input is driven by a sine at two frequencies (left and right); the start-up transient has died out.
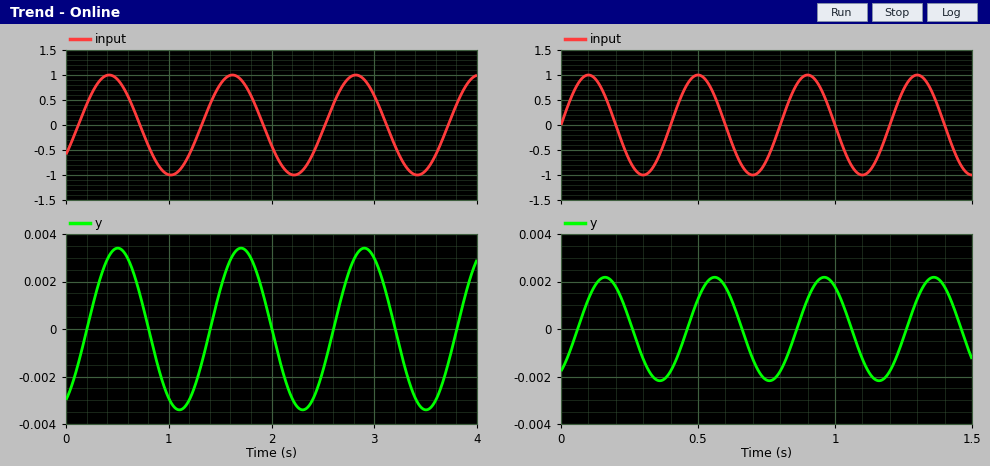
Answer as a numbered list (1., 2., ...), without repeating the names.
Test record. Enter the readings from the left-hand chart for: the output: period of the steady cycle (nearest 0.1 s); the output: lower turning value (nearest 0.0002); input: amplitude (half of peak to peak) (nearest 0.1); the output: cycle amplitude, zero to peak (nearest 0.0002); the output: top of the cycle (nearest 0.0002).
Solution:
1. 1.2 s
2. -0.0034
3. 1.0
4. 0.0034
5. 0.0034
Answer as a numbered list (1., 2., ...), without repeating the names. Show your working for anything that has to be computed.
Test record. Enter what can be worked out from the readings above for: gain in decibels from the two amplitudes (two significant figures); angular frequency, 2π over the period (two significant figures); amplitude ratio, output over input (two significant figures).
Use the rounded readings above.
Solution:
1. 20 log10(0.0034 / 1) = -49 dB
2. 2π / 1.2 = 5.2 rad/s
3. 0.0034 / 1 = 0.0034
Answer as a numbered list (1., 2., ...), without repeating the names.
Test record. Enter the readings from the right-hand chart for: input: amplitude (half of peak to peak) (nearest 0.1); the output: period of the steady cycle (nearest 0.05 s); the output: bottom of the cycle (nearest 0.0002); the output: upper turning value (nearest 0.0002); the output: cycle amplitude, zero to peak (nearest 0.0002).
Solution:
1. 1.0
2. 0.40 s
3. -0.0022
4. 0.0022
5. 0.0022
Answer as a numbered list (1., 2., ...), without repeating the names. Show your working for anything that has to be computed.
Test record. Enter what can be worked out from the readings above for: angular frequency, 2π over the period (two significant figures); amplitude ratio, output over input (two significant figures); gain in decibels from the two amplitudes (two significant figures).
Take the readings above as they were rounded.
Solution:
1. 2π / 0.4 = 16 rad/s
2. 0.0022 / 1 = 0.0022
3. 20 log10(0.0022 / 1) = -53 dB
